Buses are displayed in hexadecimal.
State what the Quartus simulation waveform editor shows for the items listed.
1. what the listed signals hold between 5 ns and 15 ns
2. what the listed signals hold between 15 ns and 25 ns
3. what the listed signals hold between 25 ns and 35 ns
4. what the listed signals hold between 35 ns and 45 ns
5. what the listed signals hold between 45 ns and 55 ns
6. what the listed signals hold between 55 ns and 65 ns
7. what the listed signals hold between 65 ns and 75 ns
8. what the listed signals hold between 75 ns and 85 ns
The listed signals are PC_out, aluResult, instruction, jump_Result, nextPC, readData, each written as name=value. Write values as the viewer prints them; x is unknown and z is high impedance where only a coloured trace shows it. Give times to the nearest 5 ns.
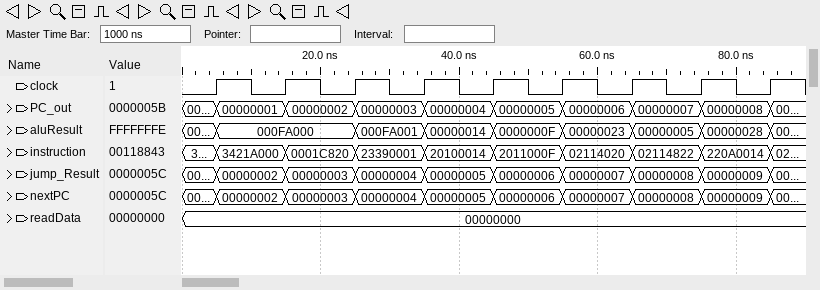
PC_out=00000001, aluResult=000FA000, instruction=3421A000, jump_Result=00000002, nextPC=00000002, readData=00000000
PC_out=00000002, aluResult=000FA000, instruction=0001C820, jump_Result=00000003, nextPC=00000003, readData=00000000
PC_out=00000003, aluResult=000FA001, instruction=23390001, jump_Result=00000004, nextPC=00000004, readData=00000000
PC_out=00000004, aluResult=00000014, instruction=20100014, jump_Result=00000005, nextPC=00000005, readData=00000000
PC_out=00000005, aluResult=0000000F, instruction=2011000F, jump_Result=00000006, nextPC=00000006, readData=00000000
PC_out=00000006, aluResult=00000023, instruction=02114020, jump_Result=00000007, nextPC=00000007, readData=00000000
PC_out=00000007, aluResult=00000005, instruction=02114822, jump_Result=00000008, nextPC=00000008, readData=00000000
PC_out=00000008, aluResult=00000028, instruction=220A0014, jump_Result=00000009, nextPC=00000009, readData=00000000
